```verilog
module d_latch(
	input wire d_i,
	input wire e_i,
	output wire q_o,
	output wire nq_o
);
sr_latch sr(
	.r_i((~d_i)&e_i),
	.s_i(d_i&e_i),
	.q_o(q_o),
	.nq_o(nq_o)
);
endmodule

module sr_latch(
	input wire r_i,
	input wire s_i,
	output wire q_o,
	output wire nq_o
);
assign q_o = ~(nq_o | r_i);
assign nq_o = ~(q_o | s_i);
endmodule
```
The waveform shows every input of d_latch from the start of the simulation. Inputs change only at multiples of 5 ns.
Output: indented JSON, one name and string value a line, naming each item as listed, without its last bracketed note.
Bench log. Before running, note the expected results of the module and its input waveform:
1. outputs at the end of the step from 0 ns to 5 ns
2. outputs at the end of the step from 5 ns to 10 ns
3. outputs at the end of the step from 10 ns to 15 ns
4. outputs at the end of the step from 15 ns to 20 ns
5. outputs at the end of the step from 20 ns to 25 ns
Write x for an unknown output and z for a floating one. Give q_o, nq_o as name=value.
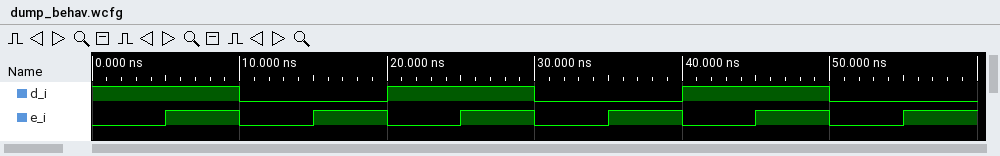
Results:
{
  "outputs at the end of the step from 0 ns to 5 ns": "q_o=x, nq_o=x",
  "outputs at the end of the step from 5 ns to 10 ns": "q_o=1, nq_o=0",
  "outputs at the end of the step from 10 ns to 15 ns": "q_o=1, nq_o=0",
  "outputs at the end of the step from 15 ns to 20 ns": "q_o=0, nq_o=1",
  "outputs at the end of the step from 20 ns to 25 ns": "q_o=0, nq_o=1"
}
